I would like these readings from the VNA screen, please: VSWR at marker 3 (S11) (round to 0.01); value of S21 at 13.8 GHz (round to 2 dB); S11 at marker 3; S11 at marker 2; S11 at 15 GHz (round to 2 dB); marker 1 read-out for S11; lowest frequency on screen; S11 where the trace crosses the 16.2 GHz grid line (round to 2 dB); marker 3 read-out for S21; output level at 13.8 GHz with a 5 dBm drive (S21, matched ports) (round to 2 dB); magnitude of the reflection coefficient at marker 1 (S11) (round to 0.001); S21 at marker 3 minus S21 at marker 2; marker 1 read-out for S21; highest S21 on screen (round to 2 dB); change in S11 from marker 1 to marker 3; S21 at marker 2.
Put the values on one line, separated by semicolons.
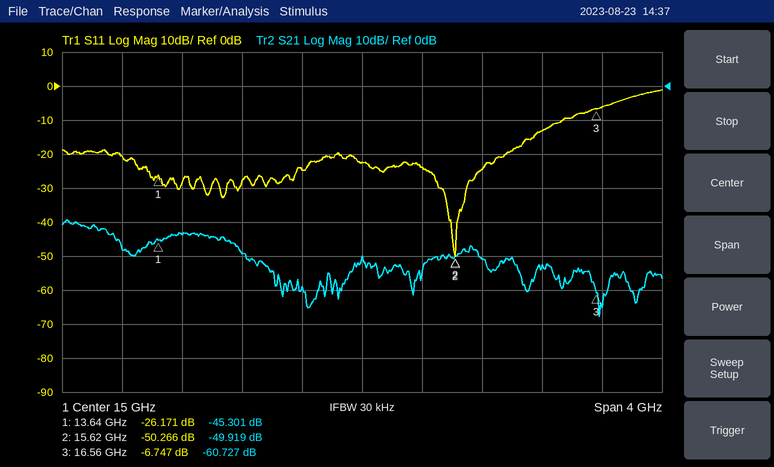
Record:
2.70; -44 dB; -6.747 dB; -50.266 dB; -22 dB; -26.171 dB; 13 GHz; -14 dB; -60.727 dB; -38 dBm; 0.049; -10.808 dB; -45.301 dB; -40 dB; 19.424 dB; -49.919 dB
